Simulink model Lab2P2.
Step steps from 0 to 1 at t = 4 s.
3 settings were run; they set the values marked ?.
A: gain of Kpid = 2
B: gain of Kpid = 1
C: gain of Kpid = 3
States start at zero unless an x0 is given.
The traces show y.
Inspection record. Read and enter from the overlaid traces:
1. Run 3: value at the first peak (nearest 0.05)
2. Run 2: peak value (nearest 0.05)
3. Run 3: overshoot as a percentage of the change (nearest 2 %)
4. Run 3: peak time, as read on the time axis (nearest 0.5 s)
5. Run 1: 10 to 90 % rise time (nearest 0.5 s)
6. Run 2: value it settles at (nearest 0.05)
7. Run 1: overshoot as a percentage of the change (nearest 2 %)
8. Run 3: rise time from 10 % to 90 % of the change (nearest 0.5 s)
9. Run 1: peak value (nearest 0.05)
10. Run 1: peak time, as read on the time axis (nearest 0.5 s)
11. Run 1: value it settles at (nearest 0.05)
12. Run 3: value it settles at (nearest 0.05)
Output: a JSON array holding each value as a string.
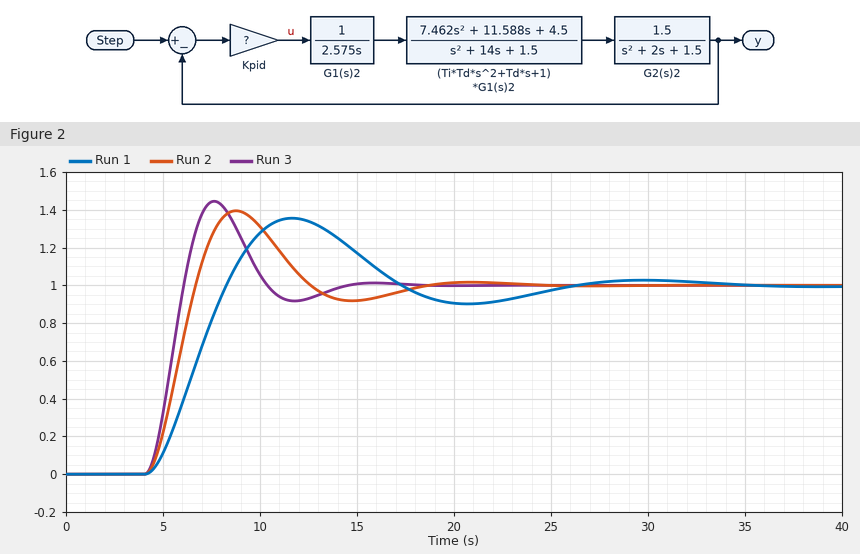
["1.45", "1.40", "44 %", "7.5 s", "3.0 s", "1.00", "36 %", "1.5 s", "1.35", "11.5 s", "1.00", "1.00"]
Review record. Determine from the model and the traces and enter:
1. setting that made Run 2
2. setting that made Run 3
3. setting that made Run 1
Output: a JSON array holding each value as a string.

["A", "C", "B"]
